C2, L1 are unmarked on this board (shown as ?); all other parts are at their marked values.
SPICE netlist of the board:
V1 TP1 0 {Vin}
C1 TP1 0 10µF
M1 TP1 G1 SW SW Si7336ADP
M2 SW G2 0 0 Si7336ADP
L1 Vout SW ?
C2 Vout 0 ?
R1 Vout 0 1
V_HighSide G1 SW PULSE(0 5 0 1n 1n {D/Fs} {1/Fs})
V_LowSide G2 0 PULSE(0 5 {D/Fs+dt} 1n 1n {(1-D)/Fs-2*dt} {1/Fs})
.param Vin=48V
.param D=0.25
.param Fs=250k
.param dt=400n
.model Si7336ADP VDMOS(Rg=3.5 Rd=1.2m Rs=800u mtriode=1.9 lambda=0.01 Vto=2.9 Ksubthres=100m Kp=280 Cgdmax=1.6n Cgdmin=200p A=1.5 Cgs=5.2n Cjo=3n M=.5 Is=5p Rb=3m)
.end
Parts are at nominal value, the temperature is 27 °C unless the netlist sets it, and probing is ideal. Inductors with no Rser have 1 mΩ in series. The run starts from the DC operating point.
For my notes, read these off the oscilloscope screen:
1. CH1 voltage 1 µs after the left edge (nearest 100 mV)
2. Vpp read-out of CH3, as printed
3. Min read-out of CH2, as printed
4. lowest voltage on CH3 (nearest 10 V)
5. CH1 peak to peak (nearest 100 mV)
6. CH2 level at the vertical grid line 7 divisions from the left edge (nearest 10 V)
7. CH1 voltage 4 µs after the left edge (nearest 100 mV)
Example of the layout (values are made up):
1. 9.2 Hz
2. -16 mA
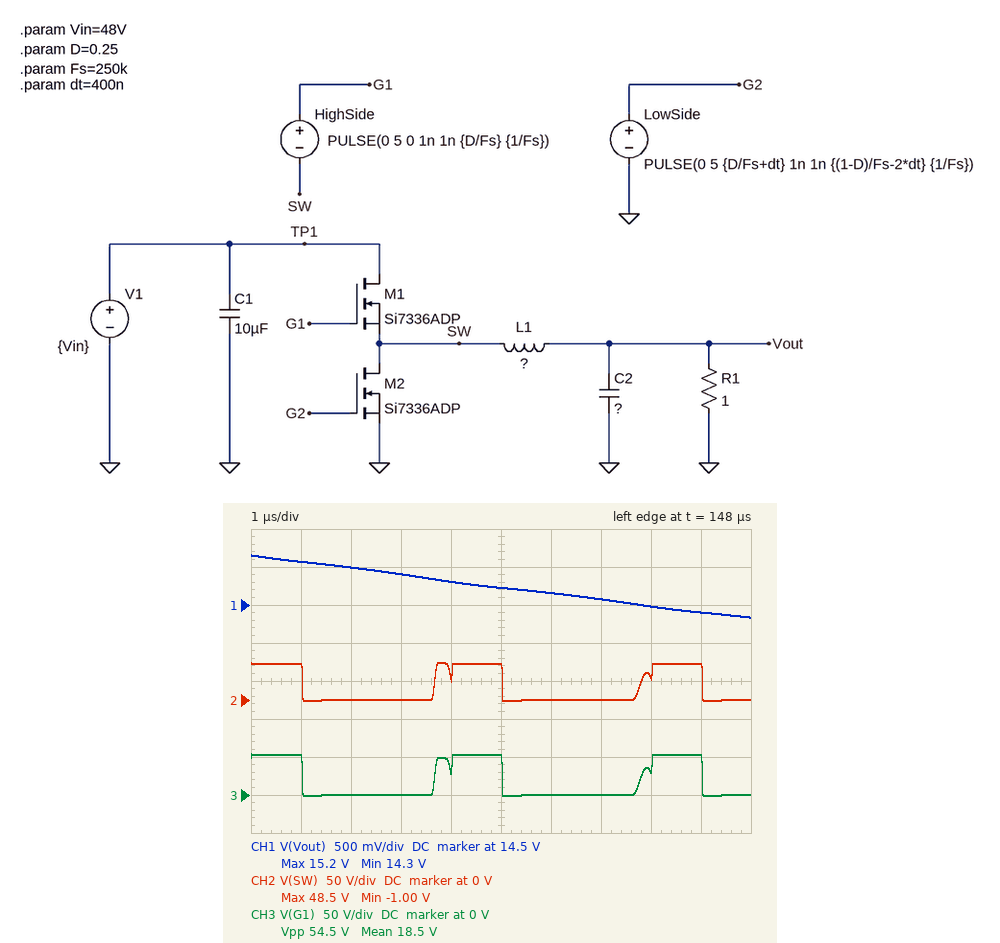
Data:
1. 15.1 V
2. 54.5 V
3. -1.00 V
4. 0 V
5. 800 mV
6. 0 V
7. 14.8 V
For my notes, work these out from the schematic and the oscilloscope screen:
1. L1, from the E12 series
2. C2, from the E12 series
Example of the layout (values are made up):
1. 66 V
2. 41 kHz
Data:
1. 6.8 µH
2. 150 µF
